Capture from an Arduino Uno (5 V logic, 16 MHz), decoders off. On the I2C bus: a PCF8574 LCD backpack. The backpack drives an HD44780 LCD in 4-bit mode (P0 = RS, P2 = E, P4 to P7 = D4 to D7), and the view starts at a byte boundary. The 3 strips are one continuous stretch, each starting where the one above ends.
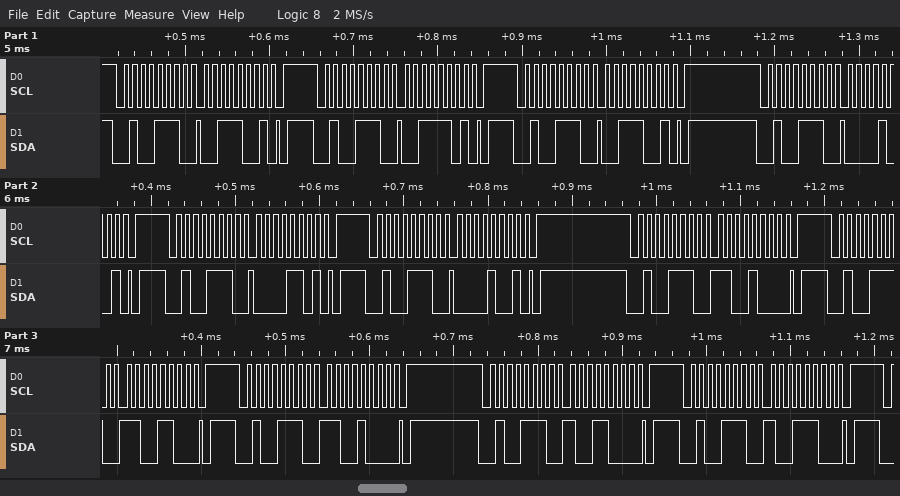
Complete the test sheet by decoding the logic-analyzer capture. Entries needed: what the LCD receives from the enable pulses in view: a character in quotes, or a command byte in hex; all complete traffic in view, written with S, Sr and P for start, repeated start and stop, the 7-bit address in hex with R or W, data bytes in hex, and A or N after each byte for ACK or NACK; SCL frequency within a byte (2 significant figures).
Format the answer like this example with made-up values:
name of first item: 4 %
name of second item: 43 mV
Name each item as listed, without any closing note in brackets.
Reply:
what the LCD receives from the enable pulses in view: a character in quotes, or a command byte in hex: '0'
all complete traffic in view, written with S, Sr and P for start, repeated start and stop, the 7-bit address in hex with R or W, data bytes in hex, and A or N after each byte for ACK or NACK: S 27W A 39 A P S 27W A 3D A P S 27W A 39 A P S 27W A 09 A P S 27W A 0D A P S 27W A 09 A P S 27W A C8 A P S 27W A CC A P S 27W A C8 A P S 27W A 98 A P S 27W A 9C A P
SCL frequency within a byte: 100 kHz
